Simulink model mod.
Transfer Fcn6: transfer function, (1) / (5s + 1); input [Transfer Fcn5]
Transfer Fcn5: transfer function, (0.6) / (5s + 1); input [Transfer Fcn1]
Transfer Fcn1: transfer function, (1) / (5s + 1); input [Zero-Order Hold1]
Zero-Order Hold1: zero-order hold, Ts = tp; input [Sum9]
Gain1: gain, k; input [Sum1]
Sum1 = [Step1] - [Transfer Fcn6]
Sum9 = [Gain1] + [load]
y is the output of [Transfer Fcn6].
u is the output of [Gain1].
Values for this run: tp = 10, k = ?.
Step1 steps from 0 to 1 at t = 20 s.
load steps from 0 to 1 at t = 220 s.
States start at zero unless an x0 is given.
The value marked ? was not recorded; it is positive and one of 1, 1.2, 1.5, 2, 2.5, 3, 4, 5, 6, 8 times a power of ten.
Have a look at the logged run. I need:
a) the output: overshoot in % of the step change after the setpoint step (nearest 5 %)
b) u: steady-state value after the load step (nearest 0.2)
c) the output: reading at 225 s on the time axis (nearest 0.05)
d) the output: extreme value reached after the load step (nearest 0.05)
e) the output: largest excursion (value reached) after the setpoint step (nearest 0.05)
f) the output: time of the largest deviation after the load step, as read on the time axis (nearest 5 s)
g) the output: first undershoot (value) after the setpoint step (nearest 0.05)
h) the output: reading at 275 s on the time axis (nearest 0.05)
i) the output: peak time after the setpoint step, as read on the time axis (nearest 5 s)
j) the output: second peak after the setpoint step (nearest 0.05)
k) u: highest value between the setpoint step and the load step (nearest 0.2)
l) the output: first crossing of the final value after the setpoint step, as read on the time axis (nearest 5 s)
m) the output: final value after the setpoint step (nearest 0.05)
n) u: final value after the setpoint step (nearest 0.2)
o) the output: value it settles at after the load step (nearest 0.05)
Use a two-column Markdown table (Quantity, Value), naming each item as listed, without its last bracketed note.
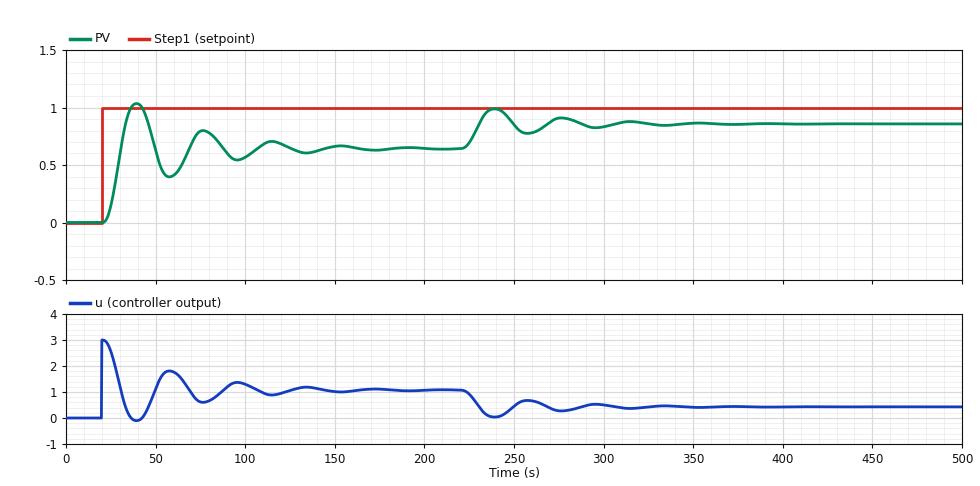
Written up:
| Quantity | Value |
|---|---|
| the output: overshoot in % of the step change after the setpoint step | 60 % |
| u: steady-state value after the load step | 0.4 |
| the output: reading at 225 s on the time axis | 0.70 |
| the output: extreme value reached after the load step | 1.00 |
| the output: largest excursion (value reached) after the setpoint step | 1.05 |
| the output: time of the largest deviation after the load step, as read on the time axis | 240 s |
| the output: first undershoot (value) after the setpoint step | 0.40 |
| the output: reading at 275 s on the time axis | 0.90 |
| the output: peak time after the setpoint step, as read on the time axis | 40 s |
| the output: second peak after the setpoint step | 0.80 |
| u: highest value between the setpoint step and the load step | 3.0 |
| the output: first crossing of the final value after the setpoint step, as read on the time axis | 30 s |
| the output: final value after the setpoint step | 0.65 |
| u: final value after the setpoint step | 1.0 |
| the output: value it settles at after the load step | 0.85 |
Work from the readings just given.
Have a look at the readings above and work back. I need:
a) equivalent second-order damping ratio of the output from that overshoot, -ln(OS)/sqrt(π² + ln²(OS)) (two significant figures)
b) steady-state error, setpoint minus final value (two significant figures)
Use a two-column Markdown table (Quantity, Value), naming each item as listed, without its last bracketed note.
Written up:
| Quantity | Value |
|---|---|
| equivalent second-order damping ratio of the output from that overshoot, -ln(OS)/sqrt(π² + ln²(OS)) | 0.16 |
| steady-state error, setpoint minus final value | 0.35 |
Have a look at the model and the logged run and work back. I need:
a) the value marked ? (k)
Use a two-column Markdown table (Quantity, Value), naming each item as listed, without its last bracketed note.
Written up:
| Quantity | Value |
|---|---|
| the value marked ? | 3 |
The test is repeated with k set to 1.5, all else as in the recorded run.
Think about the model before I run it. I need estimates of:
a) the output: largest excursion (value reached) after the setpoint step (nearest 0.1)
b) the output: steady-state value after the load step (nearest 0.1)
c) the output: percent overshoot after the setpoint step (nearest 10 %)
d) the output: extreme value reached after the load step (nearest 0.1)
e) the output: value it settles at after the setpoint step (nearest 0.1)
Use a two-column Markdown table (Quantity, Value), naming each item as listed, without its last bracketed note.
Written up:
| Quantity | Value |
|---|---|
| the output: largest excursion (value reached) after the setpoint step | 0.6 |
| the output: steady-state value after the load step | 0.8 |
| the output: percent overshoot after the setpoint step | 30 % |
| the output: extreme value reached after the load step | 0.9 |
| the output: value it settles at after the setpoint step | 0.5 |
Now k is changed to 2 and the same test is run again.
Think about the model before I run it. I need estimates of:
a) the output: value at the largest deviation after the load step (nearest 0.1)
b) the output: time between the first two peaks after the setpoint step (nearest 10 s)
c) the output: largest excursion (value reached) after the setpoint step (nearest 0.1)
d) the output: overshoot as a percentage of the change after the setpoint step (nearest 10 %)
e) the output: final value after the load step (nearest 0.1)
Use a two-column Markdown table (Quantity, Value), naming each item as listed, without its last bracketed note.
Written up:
| Quantity | Value |
|---|---|
| the output: value at the largest deviation after the load step | 0.9 |
| the output: time between the first two peaks after the setpoint step | 40 s |
| the output: largest excursion (value reached) after the setpoint step | 0.8 |
| the output: overshoot as a percentage of the change after the setpoint step | 40 % |
| the output: final value after the load step | 0.8 |
